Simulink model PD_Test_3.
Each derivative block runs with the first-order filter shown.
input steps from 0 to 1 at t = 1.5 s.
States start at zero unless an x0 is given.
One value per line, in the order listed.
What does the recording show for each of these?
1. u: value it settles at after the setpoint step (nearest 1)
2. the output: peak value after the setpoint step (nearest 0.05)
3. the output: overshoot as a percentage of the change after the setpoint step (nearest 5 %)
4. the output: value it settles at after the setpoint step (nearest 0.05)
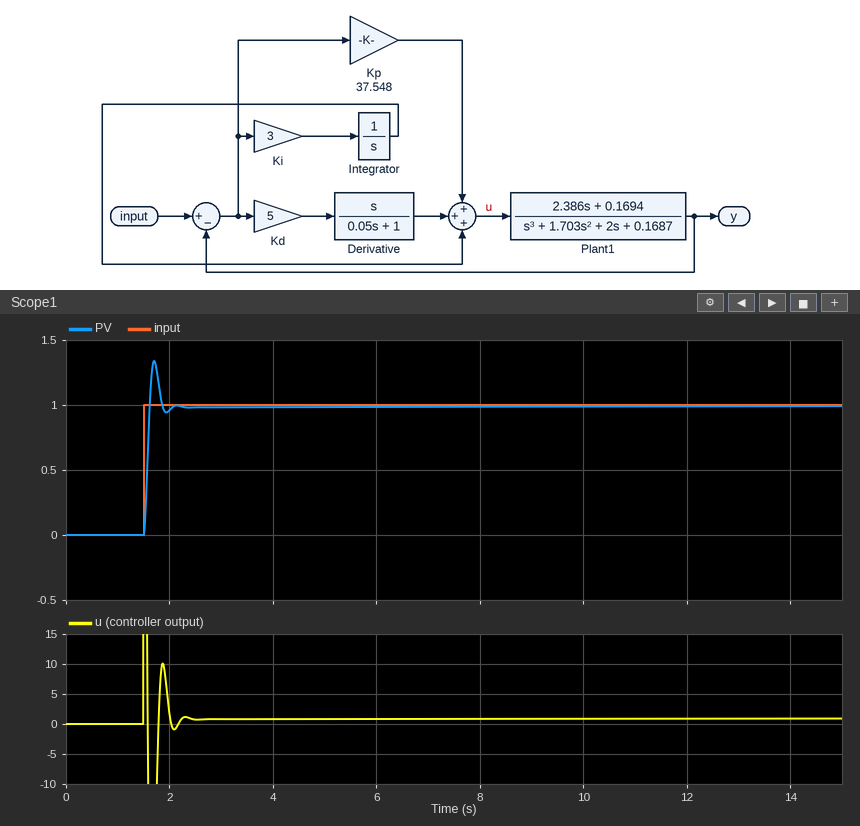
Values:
1
1.35
35 %
1.00
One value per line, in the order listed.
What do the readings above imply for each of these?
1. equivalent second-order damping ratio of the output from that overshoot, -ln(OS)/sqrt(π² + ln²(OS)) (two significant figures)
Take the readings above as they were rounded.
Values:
0.32
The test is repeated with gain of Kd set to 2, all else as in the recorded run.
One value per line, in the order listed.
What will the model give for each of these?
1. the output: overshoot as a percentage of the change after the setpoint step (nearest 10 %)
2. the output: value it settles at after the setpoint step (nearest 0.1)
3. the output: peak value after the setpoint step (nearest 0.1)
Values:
50 %
1.0
1.5
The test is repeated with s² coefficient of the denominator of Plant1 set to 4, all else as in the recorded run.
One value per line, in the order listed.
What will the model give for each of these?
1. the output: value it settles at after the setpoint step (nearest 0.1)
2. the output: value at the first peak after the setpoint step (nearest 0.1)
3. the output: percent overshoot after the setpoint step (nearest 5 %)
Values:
1.0
1.2
20 %
